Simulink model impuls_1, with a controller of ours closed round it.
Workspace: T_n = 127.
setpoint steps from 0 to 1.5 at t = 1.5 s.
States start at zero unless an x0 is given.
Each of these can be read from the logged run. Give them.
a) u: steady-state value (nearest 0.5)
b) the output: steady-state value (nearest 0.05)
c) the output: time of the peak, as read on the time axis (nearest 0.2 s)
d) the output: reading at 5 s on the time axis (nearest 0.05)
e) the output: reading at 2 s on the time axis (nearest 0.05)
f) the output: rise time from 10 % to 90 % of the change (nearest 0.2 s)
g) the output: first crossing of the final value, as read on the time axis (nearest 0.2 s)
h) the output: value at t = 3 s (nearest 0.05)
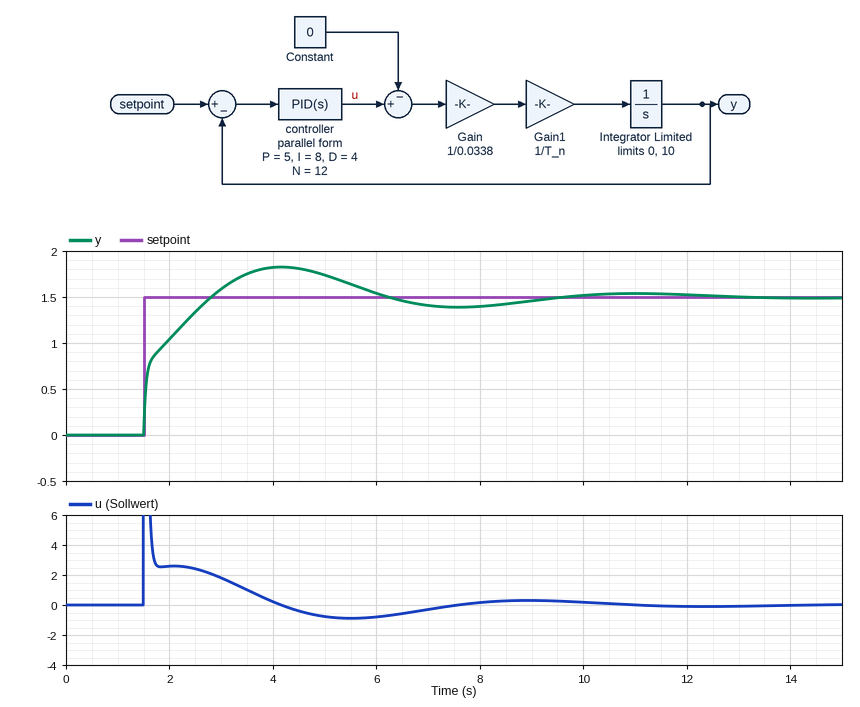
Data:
0.0
1.50
4.2 s
1.75
1.05
1.0 s
2.8 s
1.60
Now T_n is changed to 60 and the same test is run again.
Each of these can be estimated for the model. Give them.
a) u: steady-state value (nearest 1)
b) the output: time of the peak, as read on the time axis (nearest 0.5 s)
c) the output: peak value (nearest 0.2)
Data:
0
3.5 s
1.6
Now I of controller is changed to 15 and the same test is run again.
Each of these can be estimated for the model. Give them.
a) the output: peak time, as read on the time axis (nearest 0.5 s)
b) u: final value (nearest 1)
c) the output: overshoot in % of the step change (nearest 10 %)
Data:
3.5 s
0
30 %
